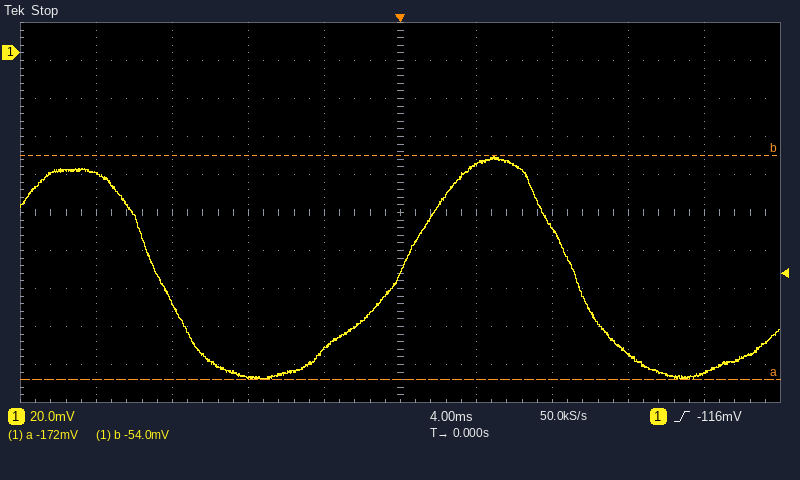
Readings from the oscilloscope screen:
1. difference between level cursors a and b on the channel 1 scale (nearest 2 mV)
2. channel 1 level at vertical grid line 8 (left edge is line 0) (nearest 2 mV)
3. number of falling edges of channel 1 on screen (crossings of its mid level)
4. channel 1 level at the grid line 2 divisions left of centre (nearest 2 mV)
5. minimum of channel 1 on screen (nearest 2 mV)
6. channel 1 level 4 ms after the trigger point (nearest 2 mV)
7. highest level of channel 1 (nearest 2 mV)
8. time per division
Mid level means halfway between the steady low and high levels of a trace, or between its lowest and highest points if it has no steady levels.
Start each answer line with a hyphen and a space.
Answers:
- 118 mV
- -158 mV
- 2
- -170 mV
- -172 mV
- -58 mV
- -54 mV
- 4 ms
